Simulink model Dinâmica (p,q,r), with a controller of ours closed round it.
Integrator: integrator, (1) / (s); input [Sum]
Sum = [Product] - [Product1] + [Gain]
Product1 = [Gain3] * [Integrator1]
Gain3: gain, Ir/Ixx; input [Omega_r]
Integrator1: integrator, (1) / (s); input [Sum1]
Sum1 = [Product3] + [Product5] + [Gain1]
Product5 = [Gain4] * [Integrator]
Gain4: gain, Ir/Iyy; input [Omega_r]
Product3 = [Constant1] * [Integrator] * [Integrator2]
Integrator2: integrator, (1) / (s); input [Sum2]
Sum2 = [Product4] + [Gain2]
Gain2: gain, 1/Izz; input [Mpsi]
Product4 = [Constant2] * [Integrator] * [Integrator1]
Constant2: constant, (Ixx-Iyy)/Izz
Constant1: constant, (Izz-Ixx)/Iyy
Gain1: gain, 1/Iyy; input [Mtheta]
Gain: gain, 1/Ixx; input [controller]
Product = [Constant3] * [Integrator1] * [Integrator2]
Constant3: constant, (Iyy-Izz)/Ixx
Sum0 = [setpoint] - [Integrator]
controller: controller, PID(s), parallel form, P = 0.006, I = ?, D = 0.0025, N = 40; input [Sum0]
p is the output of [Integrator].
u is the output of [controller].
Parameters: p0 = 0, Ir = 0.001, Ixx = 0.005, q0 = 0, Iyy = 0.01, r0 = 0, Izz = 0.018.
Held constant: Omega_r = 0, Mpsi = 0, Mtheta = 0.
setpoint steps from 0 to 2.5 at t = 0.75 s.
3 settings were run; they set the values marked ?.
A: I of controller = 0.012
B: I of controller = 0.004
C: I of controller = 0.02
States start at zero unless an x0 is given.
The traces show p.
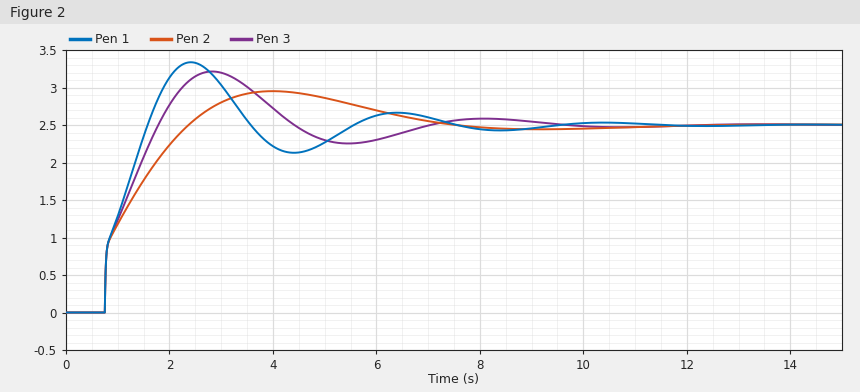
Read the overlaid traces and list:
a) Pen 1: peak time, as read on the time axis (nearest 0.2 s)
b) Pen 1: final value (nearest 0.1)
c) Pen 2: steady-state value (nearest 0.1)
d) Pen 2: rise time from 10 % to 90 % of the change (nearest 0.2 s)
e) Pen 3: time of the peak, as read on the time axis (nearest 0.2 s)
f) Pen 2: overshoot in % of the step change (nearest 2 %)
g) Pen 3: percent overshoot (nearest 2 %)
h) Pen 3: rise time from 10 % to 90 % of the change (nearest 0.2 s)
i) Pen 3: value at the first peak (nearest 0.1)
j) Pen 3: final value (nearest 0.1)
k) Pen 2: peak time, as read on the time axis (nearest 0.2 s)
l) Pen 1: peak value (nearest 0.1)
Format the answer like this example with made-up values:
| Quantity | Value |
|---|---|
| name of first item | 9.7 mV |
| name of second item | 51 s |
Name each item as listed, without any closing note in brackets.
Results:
| Quantity | Value |
|---|---|
| Pen 1: peak time, as read on the time axis | 2.4 s |
| Pen 1: final value | 2.5 |
| Pen 2: steady-state value | 2.5 |
| Pen 2: rise time from 10 % to 90 % of the change | 1.2 s |
| Pen 3: time of the peak, as read on the time axis | 2.8 s |
| Pen 2: overshoot in % of the step change | 18 % |
| Pen 3: percent overshoot | 28 % |
| Pen 3: rise time from 10 % to 90 % of the change | 0.8 s |
| Pen 3: value at the first peak | 3.2 |
| Pen 3: final value | 2.5 |
| Pen 2: peak time, as read on the time axis | 4.0 s |
| Pen 1: peak value | 3.3 |
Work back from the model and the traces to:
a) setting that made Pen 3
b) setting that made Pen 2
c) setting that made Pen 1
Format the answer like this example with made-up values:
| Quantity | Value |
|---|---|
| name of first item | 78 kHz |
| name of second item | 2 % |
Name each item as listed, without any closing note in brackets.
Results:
| Quantity | Value |
|---|---|
| setting that made Pen 3 | A |
| setting that made Pen 2 | B |
| setting that made Pen 1 | C |
